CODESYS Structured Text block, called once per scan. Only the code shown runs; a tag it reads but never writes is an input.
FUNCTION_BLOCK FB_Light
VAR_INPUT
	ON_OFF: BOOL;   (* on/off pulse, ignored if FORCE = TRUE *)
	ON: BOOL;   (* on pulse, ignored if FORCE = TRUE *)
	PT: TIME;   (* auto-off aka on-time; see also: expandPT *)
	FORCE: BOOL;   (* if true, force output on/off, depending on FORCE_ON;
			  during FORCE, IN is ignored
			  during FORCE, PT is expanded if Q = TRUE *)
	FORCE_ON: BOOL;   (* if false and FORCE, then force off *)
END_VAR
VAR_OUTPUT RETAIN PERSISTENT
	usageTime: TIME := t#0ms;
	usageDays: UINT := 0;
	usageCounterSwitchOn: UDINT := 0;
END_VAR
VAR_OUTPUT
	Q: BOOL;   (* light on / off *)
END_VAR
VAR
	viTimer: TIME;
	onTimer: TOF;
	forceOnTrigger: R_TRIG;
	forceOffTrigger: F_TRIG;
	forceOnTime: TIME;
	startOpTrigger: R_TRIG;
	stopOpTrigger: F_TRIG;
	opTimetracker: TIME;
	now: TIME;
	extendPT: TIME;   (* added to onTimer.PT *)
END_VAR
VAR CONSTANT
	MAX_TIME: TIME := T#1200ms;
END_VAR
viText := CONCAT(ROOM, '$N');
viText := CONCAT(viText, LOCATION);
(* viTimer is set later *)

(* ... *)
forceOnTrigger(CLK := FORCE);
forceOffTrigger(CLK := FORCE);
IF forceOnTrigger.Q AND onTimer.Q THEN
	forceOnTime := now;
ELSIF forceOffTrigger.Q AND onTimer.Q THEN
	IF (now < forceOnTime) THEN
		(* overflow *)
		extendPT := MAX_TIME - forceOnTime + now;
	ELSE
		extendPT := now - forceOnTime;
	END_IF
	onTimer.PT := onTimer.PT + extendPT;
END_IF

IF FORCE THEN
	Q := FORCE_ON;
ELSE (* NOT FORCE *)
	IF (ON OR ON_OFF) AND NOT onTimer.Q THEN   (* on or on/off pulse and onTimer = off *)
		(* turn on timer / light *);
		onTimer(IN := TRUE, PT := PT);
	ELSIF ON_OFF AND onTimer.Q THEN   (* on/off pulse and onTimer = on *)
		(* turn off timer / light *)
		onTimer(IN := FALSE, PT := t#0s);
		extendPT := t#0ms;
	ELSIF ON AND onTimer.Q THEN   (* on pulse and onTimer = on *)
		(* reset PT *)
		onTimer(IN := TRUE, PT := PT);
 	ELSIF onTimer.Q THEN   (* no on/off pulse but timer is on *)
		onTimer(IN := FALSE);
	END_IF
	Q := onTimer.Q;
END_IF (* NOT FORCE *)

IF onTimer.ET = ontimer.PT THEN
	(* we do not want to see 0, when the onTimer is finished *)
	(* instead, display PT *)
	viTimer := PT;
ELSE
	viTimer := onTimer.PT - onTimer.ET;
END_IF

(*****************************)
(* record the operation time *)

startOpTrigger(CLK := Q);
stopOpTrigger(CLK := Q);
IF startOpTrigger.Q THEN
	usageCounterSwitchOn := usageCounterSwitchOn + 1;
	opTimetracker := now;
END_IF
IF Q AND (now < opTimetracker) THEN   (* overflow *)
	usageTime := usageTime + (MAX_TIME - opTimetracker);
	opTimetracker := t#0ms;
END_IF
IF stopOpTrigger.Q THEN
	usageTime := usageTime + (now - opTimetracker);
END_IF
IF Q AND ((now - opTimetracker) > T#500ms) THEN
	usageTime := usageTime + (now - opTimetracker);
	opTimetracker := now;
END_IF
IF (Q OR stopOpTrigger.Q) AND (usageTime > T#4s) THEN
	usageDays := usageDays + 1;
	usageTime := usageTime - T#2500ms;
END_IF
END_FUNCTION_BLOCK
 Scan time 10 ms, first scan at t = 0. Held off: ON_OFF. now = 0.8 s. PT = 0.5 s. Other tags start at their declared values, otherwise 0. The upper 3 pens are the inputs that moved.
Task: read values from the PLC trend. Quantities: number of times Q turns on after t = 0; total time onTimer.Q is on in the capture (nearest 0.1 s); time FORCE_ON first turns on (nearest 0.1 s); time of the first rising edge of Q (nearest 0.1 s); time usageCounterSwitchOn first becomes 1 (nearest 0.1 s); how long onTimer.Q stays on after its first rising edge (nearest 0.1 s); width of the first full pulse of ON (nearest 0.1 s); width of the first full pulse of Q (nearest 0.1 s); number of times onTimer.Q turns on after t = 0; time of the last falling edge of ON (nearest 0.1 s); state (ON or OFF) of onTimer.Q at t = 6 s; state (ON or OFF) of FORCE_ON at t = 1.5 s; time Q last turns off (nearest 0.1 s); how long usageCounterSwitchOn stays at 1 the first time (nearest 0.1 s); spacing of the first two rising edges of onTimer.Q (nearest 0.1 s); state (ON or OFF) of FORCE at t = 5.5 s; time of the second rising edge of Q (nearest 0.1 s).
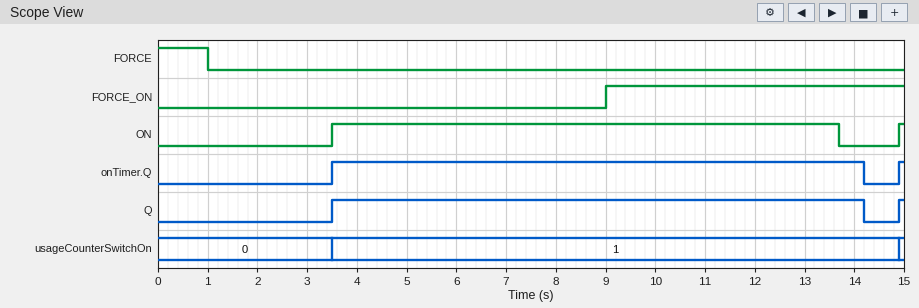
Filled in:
2
10.8 s
9.0 s
3.5 s
3.5 s
10.7 s
10.2 s
10.7 s
2
13.7 s
ON
OFF
14.2 s
11.4 s
11.4 s
OFF
14.9 s
